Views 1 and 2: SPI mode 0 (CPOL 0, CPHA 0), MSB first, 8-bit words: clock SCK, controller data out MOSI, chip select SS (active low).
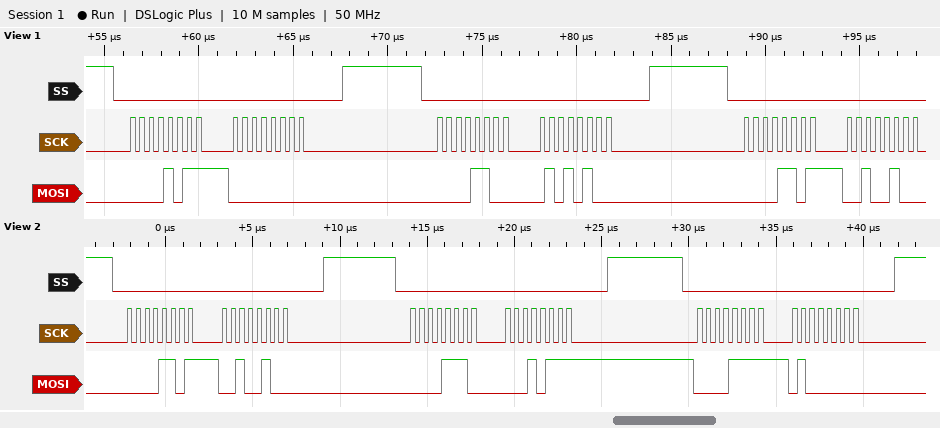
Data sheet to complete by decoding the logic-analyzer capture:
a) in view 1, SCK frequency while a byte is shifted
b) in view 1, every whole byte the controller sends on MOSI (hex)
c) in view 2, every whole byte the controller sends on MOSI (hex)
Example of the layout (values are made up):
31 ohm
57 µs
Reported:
2 MHz
0B 00 0C 54 0D 24
0D 24 0E 17 0F 40
